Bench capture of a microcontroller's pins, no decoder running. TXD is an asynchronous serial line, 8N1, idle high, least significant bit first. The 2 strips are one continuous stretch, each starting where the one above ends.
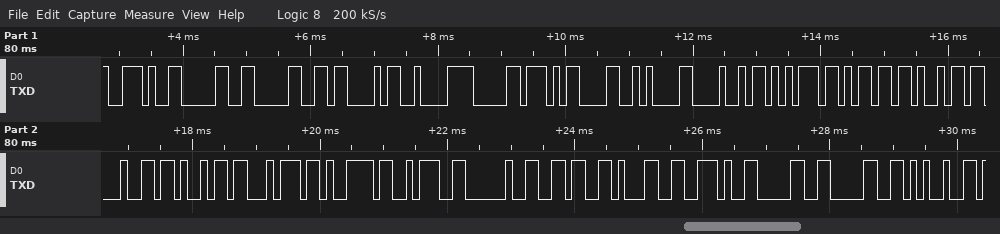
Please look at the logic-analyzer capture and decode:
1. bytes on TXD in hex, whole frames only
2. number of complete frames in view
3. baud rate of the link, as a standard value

2E 30 30 43 C2 B0 0D 0A 48 75 6D 69 64 69 74 79 3A 20 36 31 2E 30 30 25
24
9600 baud
